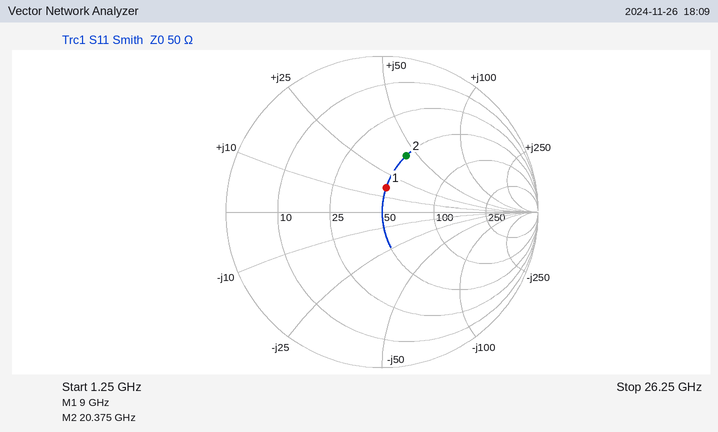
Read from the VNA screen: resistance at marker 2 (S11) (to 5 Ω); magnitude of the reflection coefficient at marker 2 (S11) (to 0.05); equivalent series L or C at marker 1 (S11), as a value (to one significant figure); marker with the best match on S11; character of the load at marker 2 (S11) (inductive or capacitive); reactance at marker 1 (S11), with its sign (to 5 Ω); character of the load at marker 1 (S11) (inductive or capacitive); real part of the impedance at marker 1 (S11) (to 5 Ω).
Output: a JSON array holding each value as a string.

["50 Ω", "0.40", "300 pH", "marker 1", "inductive", "+15 Ω", "inductive", "50 Ω"]
